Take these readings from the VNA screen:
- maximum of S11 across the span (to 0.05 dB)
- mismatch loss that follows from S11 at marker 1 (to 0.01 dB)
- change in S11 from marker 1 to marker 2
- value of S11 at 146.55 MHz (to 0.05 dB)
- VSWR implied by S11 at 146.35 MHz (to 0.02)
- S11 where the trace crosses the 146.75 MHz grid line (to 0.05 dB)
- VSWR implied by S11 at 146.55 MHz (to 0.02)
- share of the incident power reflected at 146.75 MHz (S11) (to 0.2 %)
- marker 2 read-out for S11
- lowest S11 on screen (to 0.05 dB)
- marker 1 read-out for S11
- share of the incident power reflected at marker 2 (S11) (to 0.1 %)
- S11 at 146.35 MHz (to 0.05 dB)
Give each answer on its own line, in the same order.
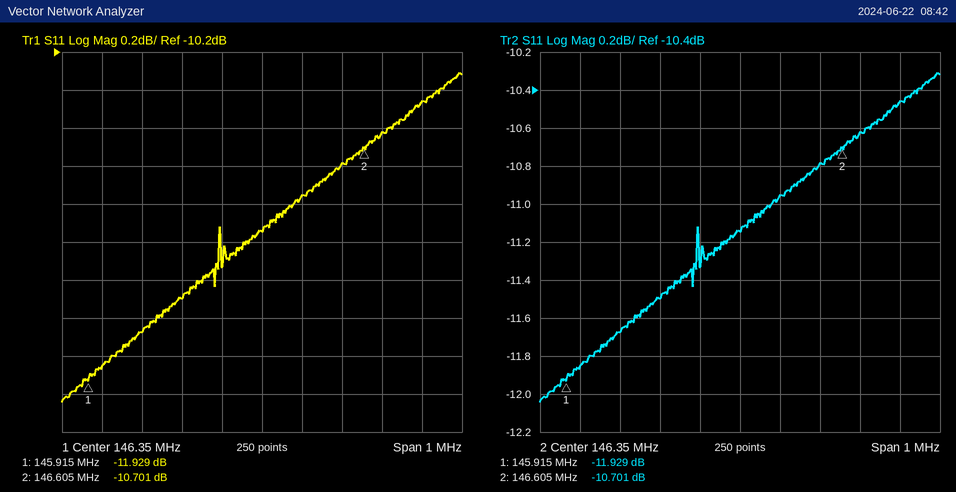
-10.30 dB
0.29 dB
1.228 dB
-10.80 dB
1.76
-10.45 dB
1.82
9.0 %
-10.701 dB
-12.05 dB
-11.929 dB
8.5 %
-11.15 dB
